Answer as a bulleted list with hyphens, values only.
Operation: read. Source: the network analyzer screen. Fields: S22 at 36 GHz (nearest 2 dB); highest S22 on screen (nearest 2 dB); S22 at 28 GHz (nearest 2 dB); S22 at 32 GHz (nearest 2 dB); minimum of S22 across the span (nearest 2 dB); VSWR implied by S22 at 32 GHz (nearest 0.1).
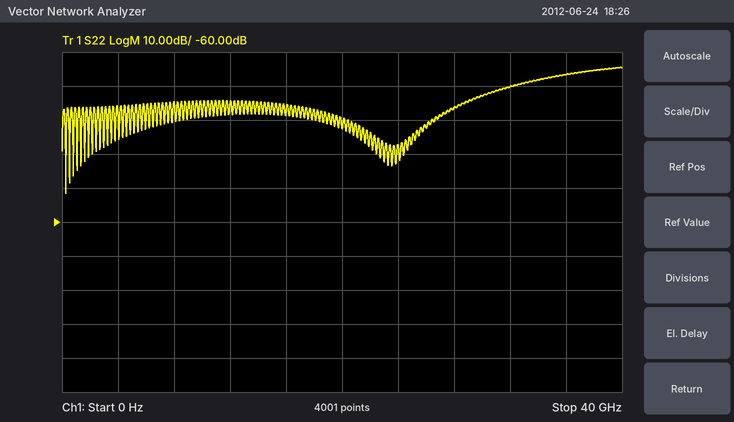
- -16 dB
- -14 dB
- -26 dB
- -20 dB
- -52 dB
- 1.2
